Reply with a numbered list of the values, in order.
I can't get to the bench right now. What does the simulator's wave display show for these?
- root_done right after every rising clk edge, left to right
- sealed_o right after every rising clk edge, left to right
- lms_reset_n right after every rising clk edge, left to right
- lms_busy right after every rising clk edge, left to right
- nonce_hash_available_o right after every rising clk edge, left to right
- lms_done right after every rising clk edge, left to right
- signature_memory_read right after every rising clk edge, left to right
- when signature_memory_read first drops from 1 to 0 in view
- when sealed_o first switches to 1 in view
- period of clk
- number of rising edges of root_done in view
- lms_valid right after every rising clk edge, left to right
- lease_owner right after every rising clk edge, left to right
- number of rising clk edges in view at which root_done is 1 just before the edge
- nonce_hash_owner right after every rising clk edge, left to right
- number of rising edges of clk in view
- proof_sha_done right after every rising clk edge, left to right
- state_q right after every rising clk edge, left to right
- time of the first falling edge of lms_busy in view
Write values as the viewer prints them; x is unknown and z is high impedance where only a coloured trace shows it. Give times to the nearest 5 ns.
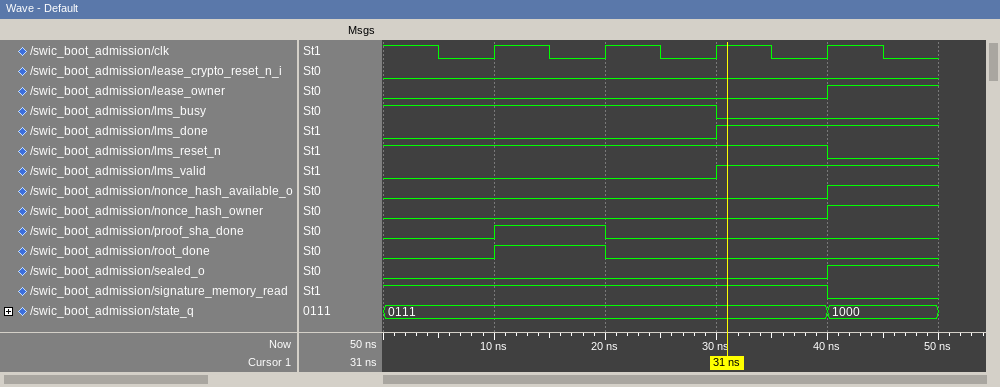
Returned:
1. 1 0 0 0
2. 0 0 0 1
3. 1 1 1 0
4. 1 1 0 0
5. 0 0 0 1
6. 0 0 1 1
7. 1 1 1 0
8. 40 ns
9. 40 ns
10. 10 ns
11. 1
12. 0 0 1 1
13. 0 0 0 1
14. 1
15. 0 0 0 1
16. 4
17. 1 0 0 0
18. 0111, 0111, 0111, 1000
19. 30 ns
